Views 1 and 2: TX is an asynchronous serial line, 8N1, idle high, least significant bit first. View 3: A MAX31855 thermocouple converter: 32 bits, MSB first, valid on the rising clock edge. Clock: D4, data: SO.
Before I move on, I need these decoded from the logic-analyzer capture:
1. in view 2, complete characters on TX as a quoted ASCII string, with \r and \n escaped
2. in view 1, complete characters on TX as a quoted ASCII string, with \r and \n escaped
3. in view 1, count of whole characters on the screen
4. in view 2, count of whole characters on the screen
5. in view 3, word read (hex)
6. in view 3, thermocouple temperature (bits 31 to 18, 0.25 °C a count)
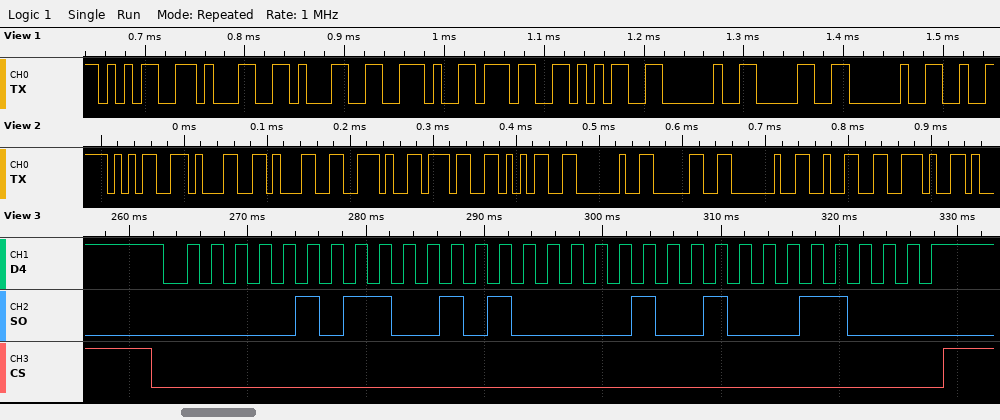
"511.75 0 2."
"511.75 0 "
9
11
0x05941230
89.25 °C
